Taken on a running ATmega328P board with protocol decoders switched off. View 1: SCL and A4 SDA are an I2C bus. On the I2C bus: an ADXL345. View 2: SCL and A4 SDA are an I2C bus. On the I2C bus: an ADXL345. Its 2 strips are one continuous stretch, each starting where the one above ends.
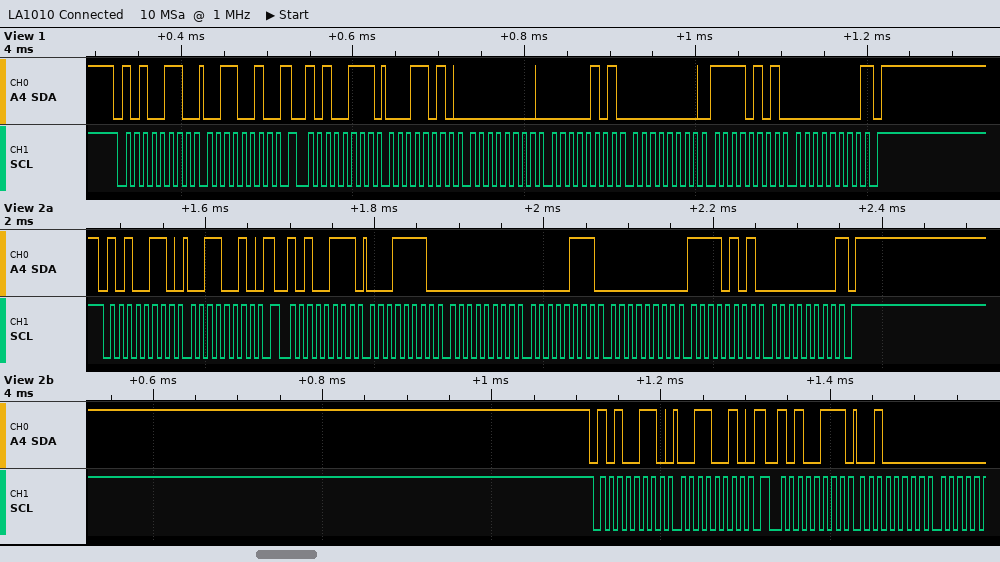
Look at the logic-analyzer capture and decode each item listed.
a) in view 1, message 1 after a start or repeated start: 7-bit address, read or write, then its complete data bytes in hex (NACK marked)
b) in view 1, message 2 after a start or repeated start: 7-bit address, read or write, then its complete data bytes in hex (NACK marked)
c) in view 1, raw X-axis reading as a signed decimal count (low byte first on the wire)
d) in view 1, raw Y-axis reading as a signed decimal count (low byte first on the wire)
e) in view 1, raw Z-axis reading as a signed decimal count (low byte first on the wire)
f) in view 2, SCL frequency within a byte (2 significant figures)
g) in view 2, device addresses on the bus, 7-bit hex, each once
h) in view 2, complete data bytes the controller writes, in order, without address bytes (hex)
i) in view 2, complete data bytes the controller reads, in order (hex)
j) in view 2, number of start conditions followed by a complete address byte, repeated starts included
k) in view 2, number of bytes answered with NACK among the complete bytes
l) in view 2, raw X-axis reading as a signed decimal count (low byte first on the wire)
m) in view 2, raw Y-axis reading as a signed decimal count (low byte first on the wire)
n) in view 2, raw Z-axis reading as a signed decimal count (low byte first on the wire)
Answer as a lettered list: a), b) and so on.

a) 0x53 write: 32
b) 0x53 read: 1A 00 05 00 F5 00 NACK
c) 26
d) 5
e) 245
f) 100 kHz
g) 0x53
h) 32 32
i) 1E 00 07 00 F5 00 20
j) 4
k) 1
l) 30
m) 7
n) 245
